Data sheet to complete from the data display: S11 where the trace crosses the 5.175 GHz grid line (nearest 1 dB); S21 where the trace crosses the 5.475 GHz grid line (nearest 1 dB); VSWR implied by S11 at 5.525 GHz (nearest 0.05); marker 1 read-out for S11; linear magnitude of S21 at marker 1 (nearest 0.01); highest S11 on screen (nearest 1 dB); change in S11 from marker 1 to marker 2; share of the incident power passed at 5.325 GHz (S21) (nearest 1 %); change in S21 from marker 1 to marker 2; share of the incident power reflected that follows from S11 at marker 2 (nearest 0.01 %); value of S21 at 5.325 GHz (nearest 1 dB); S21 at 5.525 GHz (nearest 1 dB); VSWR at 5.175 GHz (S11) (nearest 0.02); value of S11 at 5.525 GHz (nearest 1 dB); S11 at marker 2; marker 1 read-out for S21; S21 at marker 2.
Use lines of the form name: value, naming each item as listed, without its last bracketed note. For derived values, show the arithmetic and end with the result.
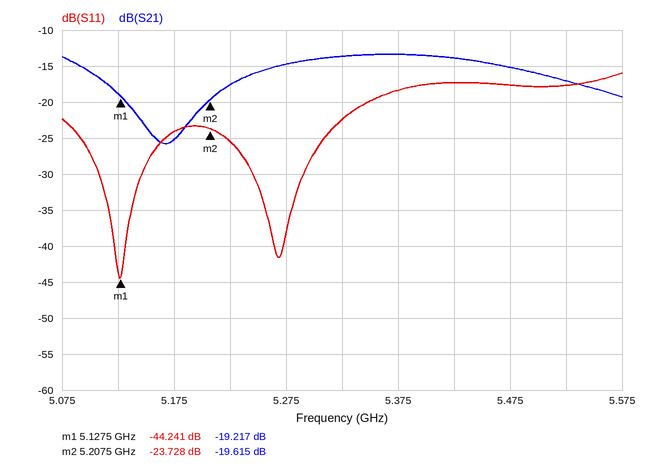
S11 where the trace crosses the 5.175 GHz grid line: -24 dB
S21 where the trace crosses the 5.475 GHz grid line: -15 dB
VSWR implied by S11 at 5.525 GHz: |Γ| = 10^(-18/20) = 0.1259; VSWR = (1 + 0.1259)/(1 − 0.1259) ≈ 1.29, so 1.30 to the nearest 0.05
marker 1 read-out for S11: -44.241 dB
linear magnitude of S21 at marker 1: 10^(-19.217/20) ≈ 0.11
highest S11 on screen: -16 dB
change in S11 from marker 1 to marker 2: -23.728 − (-44.241) = 20.513 dB
share of the incident power passed at 5.325 GHz (S21): 10^(-14/10) ≈ 4 %
change in S21 from marker 1 to marker 2: -19.615 − (-19.217) = -0.398 dB
share of the incident power reflected that follows from S11 at marker 2: 10^(-23.728/10) ≈ 0.42 %
value of S21 at 5.325 GHz: -14 dB
S21 at 5.525 GHz: -17 dB
VSWR at 5.175 GHz (S11): |Γ| = 10^(-24/20) = 0.0631; VSWR = (1 + 0.0631)/(1 − 0.0631) ≈ 1.13, so 1.14 to the nearest 0.02
value of S11 at 5.525 GHz: -18 dB
S11 at marker 2: -23.728 dB
marker 1 read-out for S21: -19.217 dB
S21 at marker 2: -19.615 dB
